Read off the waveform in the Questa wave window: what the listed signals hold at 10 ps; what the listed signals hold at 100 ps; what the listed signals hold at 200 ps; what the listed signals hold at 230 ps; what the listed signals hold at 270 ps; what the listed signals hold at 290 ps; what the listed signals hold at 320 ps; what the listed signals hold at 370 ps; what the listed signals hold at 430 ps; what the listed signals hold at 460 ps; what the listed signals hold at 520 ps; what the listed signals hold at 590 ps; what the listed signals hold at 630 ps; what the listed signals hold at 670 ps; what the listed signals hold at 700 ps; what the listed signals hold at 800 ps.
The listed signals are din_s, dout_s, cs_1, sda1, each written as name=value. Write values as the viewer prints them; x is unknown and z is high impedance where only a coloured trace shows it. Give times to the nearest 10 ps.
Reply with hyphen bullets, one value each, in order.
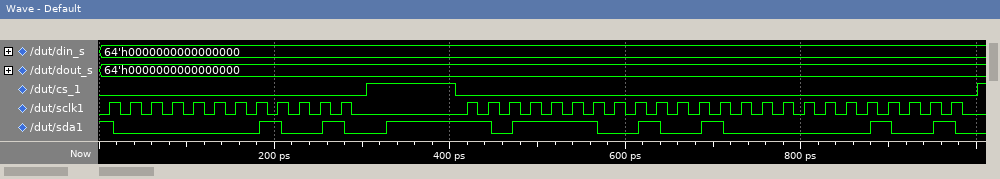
- din_s=64'h0000000000000000, dout_s=64'h0000000000000000, cs_1=0, sda1=1
- din_s=64'h0000000000000000, dout_s=64'h0000000000000000, cs_1=0, sda1=0
- din_s=64'h0000000000000000, dout_s=64'h0000000000000000, cs_1=0, sda1=1
- din_s=64'h0000000000000000, dout_s=64'h0000000000000000, cs_1=0, sda1=0
- din_s=64'h0000000000000000, dout_s=64'h0000000000000000, cs_1=0, sda1=1
- din_s=64'h0000000000000000, dout_s=64'h0000000000000000, cs_1=0, sda1=0
- din_s=64'h0000000000000000, dout_s=64'h0000000000000000, cs_1=1, sda1=0
- din_s=64'h0000000000000000, dout_s=64'h0000000000000000, cs_1=1, sda1=1
- din_s=64'h0000000000000000, dout_s=64'h0000000000000000, cs_1=0, sda1=1
- din_s=64'h0000000000000000, dout_s=64'h0000000000000000, cs_1=0, sda1=0
- din_s=64'h0000000000000000, dout_s=64'h0000000000000000, cs_1=0, sda1=1
- din_s=64'h0000000000000000, dout_s=64'h0000000000000000, cs_1=0, sda1=0
- din_s=64'h0000000000000000, dout_s=64'h0000000000000000, cs_1=0, sda1=1
- din_s=64'h0000000000000000, dout_s=64'h0000000000000000, cs_1=0, sda1=0
- din_s=64'h0000000000000000, dout_s=64'h0000000000000000, cs_1=0, sda1=1
- din_s=64'h0000000000000000, dout_s=64'h0000000000000000, cs_1=0, sda1=0
